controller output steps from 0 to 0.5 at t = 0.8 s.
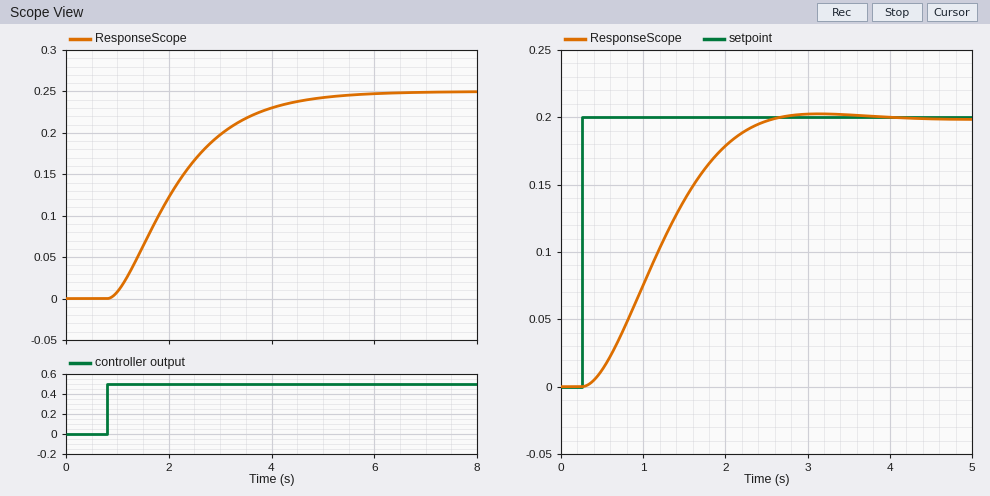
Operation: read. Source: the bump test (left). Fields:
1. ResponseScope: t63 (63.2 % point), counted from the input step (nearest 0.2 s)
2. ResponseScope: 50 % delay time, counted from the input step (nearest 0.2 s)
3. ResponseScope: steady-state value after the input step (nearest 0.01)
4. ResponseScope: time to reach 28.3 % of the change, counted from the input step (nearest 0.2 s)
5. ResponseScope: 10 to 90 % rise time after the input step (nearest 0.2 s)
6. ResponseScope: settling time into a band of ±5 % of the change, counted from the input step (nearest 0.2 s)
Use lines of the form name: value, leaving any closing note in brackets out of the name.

ResponseScope: t63 (63.2 % point), counted from the input step: 1.6 s
ResponseScope: 50 % delay time, counted from the input step: 1.2 s
ResponseScope: steady-state value after the input step: 0.25
ResponseScope: time to reach 28.3 % of the change, counted from the input step: 0.8 s
ResponseScope: 10 to 90 % rise time after the input step: 2.6 s
ResponseScope: settling time into a band of ±5 % of the change, counted from the input step: 3.6 s
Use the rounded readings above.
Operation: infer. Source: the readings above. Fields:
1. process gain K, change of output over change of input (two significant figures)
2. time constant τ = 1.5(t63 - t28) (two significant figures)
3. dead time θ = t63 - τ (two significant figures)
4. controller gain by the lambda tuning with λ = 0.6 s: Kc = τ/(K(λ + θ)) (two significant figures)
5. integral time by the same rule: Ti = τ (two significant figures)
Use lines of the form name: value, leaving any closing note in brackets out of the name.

process gain K, change of output over change of input: 0.50
time constant τ = 1.5(t63 - t28): 1.2 s
dead time θ = t63 - τ: 0.40 s
controller gain by the lambda tuning with λ = 0.6 s: Kc = τ/(K(λ + θ)): 2.4
integral time by the same rule: Ti = τ: 1.2 s
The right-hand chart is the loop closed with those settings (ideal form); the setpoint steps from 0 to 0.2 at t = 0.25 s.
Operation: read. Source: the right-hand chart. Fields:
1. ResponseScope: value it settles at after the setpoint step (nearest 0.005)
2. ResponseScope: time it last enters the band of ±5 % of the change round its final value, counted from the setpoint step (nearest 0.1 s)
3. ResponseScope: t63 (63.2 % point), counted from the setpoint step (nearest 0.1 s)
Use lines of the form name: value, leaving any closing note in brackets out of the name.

ResponseScope: value it settles at after the setpoint step: 0.200
ResponseScope: time it last enters the band of ±5 % of the change round its final value, counted from the setpoint step: 2.0 s
ResponseScope: t63 (63.2 % point), counted from the setpoint step: 1.1 s
